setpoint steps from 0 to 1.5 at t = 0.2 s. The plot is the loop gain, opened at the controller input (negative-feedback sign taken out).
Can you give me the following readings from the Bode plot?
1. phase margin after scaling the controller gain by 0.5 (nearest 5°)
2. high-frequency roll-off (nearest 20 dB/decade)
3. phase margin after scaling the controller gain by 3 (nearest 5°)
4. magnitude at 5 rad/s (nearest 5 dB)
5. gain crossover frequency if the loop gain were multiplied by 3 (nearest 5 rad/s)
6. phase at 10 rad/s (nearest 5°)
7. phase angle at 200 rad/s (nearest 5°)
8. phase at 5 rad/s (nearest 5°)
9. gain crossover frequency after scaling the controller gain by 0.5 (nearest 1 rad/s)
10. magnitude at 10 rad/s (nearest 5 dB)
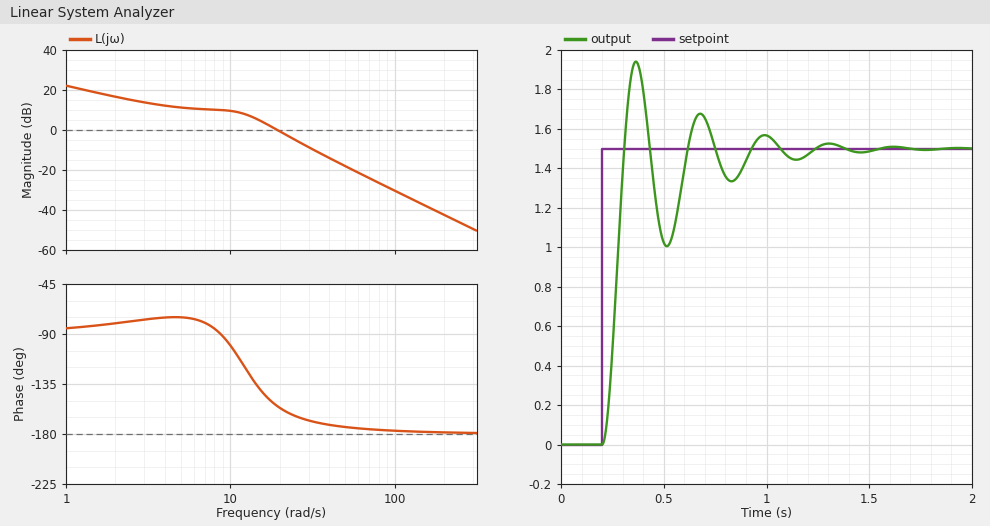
45°
-40 dB/decade
10°
10 dB
30 rad/s
-100°
-180°
-75°
14 rad/s
10 dB
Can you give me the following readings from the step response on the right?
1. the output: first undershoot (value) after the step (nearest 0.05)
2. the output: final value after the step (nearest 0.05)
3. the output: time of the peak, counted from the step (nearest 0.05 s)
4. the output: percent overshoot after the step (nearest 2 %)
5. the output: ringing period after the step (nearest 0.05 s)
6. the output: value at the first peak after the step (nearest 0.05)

1.00
1.50
0.15 s
30 %
0.30 s
1.95
